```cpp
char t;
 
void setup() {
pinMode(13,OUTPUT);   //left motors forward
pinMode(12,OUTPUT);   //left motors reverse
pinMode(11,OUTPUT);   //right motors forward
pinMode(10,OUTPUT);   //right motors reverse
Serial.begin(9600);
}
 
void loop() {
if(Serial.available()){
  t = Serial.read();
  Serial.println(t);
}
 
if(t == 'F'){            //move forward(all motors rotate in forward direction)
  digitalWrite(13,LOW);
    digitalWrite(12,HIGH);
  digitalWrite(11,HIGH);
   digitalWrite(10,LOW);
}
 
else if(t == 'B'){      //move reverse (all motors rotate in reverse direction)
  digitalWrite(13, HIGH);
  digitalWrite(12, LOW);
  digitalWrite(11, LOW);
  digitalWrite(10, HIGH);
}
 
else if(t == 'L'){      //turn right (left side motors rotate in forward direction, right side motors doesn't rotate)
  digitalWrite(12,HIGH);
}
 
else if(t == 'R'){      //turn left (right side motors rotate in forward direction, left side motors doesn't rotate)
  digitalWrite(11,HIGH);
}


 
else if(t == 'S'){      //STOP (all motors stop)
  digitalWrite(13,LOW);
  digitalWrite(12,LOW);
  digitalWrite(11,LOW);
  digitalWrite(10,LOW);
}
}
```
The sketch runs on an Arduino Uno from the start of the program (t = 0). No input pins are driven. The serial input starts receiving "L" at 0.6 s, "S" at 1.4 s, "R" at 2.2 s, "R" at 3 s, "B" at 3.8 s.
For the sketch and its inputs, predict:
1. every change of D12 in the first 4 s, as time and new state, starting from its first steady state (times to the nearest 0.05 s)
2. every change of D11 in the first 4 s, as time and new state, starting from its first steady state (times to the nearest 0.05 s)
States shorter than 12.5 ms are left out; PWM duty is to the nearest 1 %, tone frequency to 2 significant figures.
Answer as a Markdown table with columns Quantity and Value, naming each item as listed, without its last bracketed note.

| Quantity | Value |
|---|---|
| every change of D12 in the first 4 s, as time and new state, starting from its first steady state | 0 s low; 0.6 s high; 1.4 s low |
| every change of D11 in the first 4 s, as time and new state, starting from its first steady state | 0 s low; 2.2 s high; 3.8 s low |
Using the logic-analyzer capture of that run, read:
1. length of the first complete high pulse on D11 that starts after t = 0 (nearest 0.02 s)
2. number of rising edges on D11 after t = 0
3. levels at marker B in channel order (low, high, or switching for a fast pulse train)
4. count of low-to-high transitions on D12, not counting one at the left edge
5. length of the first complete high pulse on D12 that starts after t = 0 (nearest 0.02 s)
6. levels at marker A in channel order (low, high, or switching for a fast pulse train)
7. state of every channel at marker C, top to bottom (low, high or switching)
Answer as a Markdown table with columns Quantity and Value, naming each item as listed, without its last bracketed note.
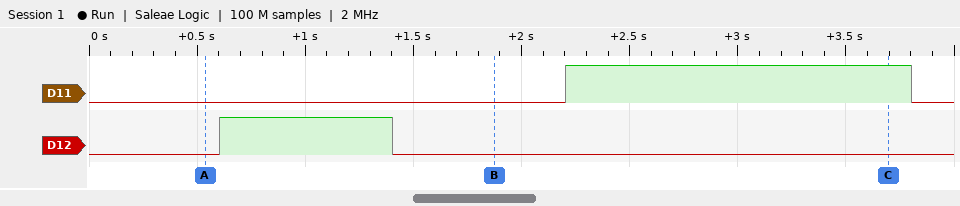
| Quantity | Value |
|---|---|
| length of the first complete high pulse on D11 that starts after t = 0 | 1.60 s |
| number of rising edges on D11 after t = 0 | 1 |
| levels at marker B in channel order | D11 low, D12 low |
| count of low-to-high transitions on D12, not counting one at the left edge | 1 |
| length of the first complete high pulse on D12 that starts after t = 0 | 0.80 s |
| levels at marker A in channel order | D11 low, D12 low |
| state of every channel at marker C, top to bottom | D11 high, D12 low |
